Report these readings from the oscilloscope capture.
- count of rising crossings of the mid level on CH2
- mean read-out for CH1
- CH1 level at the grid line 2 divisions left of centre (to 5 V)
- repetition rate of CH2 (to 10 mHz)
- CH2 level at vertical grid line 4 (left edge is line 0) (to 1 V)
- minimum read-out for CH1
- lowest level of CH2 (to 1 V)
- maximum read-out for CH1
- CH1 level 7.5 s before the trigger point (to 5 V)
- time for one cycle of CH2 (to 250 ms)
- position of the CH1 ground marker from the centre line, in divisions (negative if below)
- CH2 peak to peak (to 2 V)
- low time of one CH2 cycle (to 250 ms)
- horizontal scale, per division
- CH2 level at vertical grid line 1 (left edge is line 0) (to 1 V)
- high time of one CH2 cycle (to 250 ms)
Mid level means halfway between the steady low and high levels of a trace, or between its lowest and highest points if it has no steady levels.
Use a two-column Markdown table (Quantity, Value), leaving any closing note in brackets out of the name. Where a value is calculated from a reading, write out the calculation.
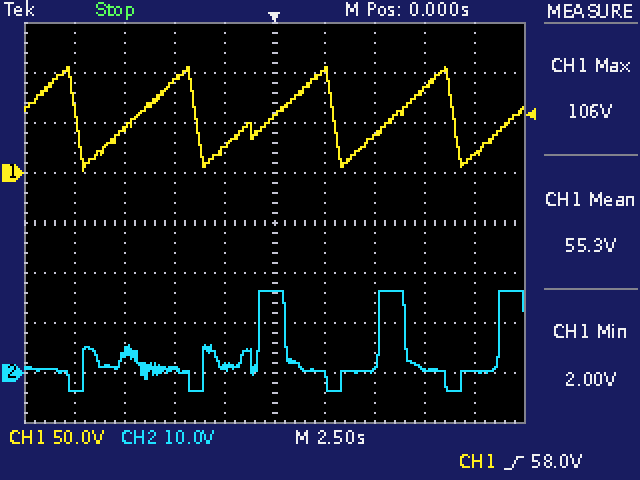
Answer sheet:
| Quantity | Value |
|---|---|
| count of rising crossings of the mid level on CH2 | 3 |
| mean read-out for CH1 | 55.3 V |
| CH1 level at the grid line 2 divisions left of centre | 95 V |
| repetition rate of CH2 | 1 / 6.00 s ≈ 167 mHz, so 170 mHz to the nearest 10 mHz |
| CH2 level at vertical grid line 4 (left edge is line 0) | 1 V |
| minimum read-out for CH1 | 2.00 V |
| lowest level of CH2 | -4 V |
| maximum read-out for CH1 | 106 V |
| CH1 level 7.5 s before the trigger point | 45 V |
| time for one cycle of CH2 | 6.00 s |
| position of the CH1 ground marker from the centre line, in divisions | +1.0 div |
| CH2 peak to peak | 20 V |
| low time of one CH2 cycle | 4.75 s |
| horizontal scale, per division | 2.5 s |
| CH2 level at vertical grid line 1 (left edge is line 0) | -4 V |
| high time of one CH2 cycle | 1.25 s |
